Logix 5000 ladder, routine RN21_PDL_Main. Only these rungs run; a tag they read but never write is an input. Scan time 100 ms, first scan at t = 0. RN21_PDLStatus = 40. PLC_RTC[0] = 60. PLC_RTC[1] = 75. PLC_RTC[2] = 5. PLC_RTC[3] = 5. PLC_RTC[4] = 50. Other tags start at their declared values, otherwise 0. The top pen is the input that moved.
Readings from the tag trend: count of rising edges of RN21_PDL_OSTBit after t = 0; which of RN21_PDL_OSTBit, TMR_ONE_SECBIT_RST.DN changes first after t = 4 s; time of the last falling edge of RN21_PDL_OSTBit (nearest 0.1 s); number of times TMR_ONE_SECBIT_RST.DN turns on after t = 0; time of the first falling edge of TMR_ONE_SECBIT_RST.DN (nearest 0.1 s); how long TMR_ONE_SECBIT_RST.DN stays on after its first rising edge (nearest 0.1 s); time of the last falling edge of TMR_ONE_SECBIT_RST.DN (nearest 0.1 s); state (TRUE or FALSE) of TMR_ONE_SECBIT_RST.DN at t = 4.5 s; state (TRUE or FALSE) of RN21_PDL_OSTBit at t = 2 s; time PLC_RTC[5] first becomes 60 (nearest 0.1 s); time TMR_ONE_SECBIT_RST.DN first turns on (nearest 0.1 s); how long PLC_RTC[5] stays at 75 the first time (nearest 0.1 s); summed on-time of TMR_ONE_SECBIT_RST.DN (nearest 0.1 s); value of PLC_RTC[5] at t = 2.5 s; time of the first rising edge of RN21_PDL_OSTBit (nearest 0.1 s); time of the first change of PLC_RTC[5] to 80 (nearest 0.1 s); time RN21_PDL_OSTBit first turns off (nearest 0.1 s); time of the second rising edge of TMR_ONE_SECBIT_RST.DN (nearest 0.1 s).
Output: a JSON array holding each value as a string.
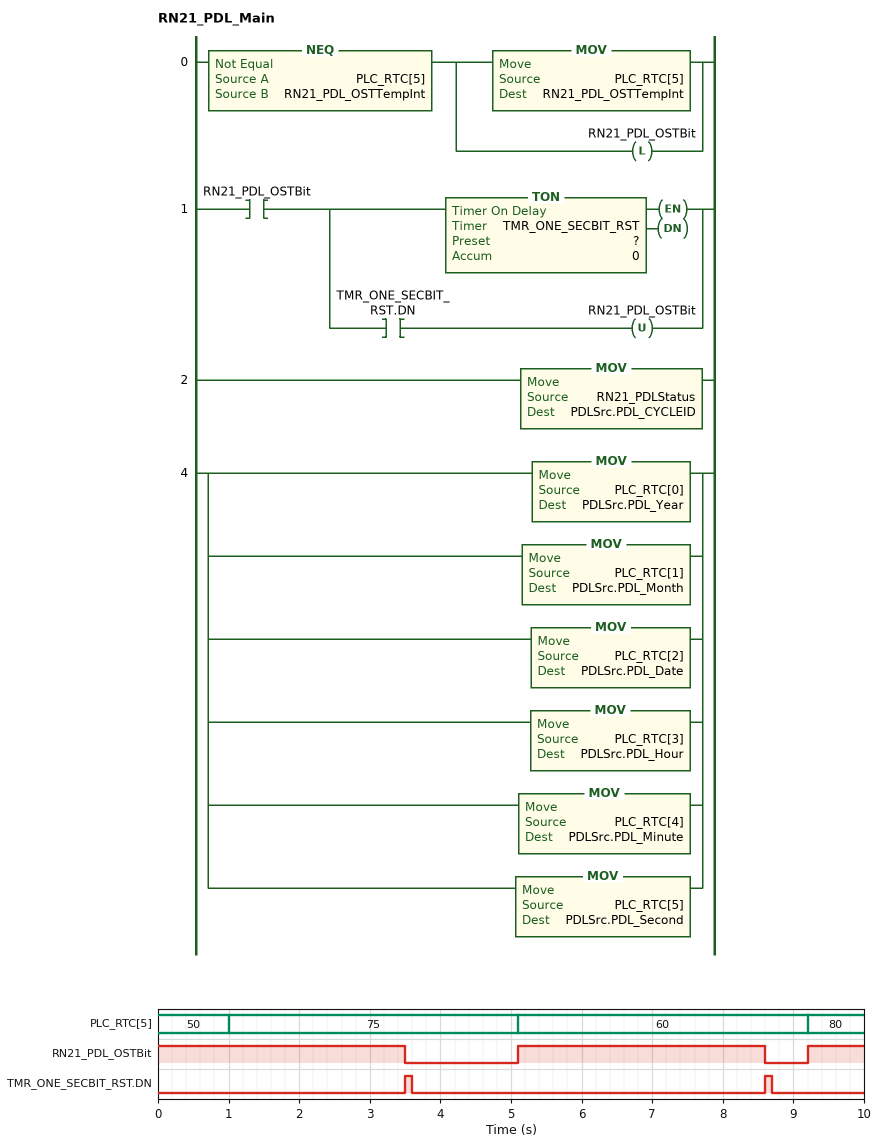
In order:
["2", "RN21_PDL_OSTBit", "8.6 s", "2", "3.6 s", "0.1 s", "8.7 s", "FALSE", "TRUE", "5.1 s", "3.5 s", "4.1 s", "0.2 s", "75", "5.1 s", "9.2 s", "3.5 s", "8.6 s"]
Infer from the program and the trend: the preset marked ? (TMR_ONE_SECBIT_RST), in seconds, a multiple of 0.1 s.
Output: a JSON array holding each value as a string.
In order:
["3.5 s"]
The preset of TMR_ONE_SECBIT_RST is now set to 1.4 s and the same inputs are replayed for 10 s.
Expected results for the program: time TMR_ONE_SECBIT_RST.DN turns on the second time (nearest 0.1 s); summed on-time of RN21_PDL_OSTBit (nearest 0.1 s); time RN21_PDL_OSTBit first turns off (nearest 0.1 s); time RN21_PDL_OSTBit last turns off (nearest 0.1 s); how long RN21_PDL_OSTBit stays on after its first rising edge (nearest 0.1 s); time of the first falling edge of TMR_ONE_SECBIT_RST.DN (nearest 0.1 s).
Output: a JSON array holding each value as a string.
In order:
["6.5 s", "3.6 s", "1.4 s", "6.5 s", "1.4 s", "1.5 s"]
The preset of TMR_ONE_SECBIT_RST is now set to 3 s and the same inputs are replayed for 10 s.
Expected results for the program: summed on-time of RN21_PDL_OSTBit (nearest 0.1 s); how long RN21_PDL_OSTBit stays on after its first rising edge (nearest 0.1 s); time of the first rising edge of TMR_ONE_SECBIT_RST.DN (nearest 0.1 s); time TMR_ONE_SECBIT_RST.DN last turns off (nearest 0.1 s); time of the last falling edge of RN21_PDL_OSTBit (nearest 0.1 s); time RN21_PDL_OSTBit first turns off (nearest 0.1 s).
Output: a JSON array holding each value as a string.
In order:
["6.8 s", "3.0 s", "3.0 s", "8.2 s", "8.1 s", "3.0 s"]
